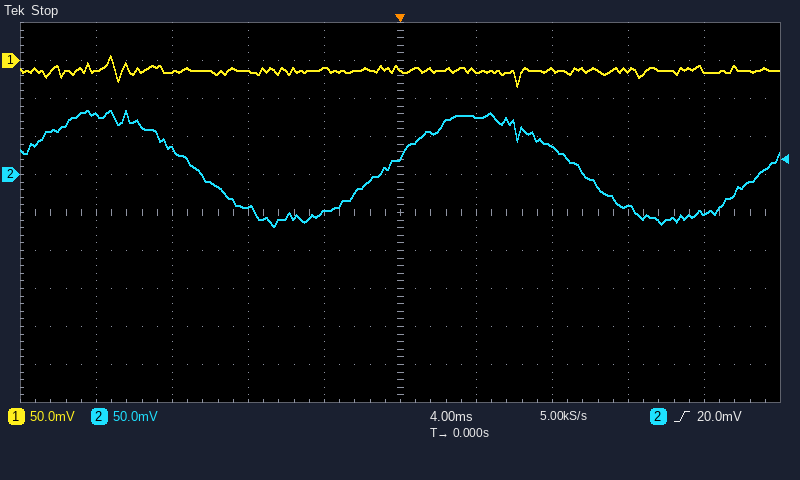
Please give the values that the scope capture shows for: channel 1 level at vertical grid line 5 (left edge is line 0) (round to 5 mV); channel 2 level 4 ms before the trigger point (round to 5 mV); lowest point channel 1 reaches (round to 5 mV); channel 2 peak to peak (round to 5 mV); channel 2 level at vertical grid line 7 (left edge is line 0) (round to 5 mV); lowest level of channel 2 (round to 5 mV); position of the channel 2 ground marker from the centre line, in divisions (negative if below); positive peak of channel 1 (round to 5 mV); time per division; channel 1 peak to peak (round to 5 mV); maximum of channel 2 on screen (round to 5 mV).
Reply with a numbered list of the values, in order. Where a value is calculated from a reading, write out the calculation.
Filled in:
1. -10 mV
2. -50 mV
3. -35 mV
4. 85 mV − (-70 mV) = 155 mV
5. 35 mV
6. -70 mV
7. +1.0 div
8. 5 mV
9. 4 ms
10. 5 mV − (-35 mV) = 40 mV
11. 85 mV
